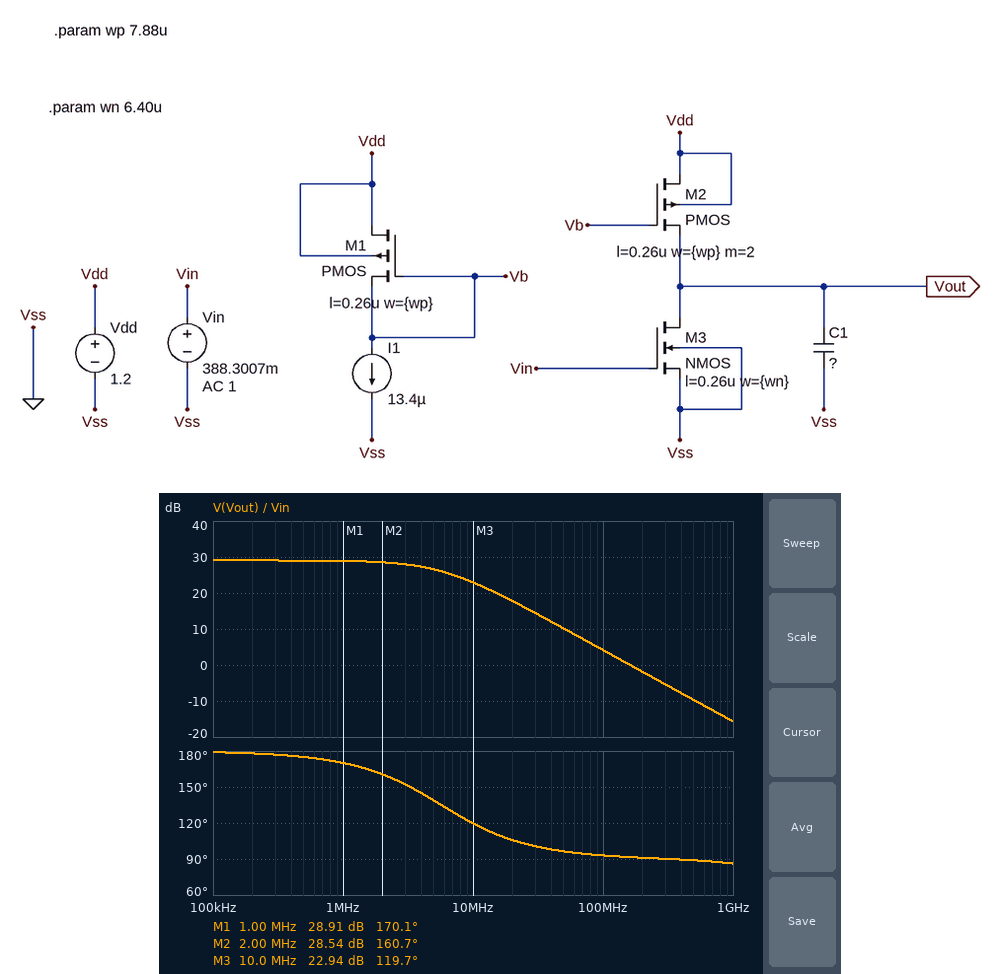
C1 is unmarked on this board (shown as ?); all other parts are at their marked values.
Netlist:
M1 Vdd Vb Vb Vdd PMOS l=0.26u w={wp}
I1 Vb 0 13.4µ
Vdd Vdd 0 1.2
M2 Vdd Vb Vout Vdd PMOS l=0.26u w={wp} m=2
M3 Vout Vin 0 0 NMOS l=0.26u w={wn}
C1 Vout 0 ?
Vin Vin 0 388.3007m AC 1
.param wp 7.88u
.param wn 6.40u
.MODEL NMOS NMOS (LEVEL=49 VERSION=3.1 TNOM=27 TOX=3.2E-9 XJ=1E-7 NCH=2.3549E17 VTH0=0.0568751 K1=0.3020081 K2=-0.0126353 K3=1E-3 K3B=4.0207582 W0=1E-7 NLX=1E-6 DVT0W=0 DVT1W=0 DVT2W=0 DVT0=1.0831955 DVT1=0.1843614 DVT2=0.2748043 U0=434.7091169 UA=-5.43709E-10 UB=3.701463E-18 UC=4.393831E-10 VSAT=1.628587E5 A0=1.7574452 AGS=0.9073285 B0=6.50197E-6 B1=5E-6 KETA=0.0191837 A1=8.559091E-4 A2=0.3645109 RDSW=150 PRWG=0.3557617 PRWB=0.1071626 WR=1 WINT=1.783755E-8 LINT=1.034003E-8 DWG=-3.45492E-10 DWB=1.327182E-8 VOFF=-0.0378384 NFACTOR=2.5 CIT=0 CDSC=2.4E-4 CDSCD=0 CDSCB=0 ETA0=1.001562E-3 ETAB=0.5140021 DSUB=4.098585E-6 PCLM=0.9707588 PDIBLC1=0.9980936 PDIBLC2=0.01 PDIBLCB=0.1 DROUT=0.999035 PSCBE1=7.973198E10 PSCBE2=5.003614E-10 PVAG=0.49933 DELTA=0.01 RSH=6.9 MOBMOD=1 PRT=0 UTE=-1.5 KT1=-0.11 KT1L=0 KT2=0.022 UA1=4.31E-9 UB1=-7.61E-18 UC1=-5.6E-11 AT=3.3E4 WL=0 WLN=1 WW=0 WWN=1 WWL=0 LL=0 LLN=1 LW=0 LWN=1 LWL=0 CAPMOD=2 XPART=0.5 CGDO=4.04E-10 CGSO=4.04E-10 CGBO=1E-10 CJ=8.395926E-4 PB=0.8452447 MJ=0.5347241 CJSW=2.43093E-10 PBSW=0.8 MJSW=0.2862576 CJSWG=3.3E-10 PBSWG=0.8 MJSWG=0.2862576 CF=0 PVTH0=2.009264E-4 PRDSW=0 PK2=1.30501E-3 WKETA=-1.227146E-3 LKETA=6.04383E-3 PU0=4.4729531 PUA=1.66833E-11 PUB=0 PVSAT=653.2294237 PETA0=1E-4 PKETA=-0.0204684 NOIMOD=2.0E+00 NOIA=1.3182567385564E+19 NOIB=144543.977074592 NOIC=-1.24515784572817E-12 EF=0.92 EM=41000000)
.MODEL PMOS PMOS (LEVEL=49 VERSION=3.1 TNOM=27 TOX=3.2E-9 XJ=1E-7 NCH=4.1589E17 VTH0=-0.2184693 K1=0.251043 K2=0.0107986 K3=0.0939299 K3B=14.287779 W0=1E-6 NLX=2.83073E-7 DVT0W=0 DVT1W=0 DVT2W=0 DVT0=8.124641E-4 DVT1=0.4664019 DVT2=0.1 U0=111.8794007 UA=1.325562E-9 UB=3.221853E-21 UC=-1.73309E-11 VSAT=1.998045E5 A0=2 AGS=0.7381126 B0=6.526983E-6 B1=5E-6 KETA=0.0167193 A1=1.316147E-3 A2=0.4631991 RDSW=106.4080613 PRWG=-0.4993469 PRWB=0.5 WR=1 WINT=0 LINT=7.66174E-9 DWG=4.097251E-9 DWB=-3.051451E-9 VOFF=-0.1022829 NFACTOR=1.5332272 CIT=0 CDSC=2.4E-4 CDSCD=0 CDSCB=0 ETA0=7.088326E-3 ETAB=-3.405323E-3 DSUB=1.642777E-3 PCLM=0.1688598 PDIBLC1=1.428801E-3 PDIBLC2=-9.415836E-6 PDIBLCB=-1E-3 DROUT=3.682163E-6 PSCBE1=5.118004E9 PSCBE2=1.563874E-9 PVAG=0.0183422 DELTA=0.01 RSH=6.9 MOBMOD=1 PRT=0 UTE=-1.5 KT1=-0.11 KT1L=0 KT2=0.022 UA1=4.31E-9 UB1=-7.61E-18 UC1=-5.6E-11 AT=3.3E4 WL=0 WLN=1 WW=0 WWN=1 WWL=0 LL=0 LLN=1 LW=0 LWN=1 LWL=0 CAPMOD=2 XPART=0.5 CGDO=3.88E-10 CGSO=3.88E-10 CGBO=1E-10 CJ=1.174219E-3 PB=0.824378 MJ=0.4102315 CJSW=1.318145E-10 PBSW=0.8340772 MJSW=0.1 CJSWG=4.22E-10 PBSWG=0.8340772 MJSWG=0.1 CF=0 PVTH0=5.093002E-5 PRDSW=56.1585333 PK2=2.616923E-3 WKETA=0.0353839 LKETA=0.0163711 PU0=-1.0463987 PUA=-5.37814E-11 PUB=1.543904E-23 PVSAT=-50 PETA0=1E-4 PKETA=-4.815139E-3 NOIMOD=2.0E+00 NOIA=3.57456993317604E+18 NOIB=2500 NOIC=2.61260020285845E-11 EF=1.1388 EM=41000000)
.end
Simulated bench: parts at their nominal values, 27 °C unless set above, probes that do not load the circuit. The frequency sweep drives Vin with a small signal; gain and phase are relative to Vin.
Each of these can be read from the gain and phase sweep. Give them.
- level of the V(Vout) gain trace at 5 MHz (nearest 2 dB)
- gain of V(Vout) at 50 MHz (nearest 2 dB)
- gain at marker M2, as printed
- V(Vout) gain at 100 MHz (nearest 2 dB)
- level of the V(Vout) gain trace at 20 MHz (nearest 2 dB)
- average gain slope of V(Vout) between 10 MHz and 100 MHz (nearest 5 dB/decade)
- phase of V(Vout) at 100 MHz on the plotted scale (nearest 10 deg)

26 dB
10 dB
28.54 dB
4 dB
18 dB
-20 dB/decade
90 deg
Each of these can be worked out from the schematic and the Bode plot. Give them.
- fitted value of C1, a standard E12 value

560 fF
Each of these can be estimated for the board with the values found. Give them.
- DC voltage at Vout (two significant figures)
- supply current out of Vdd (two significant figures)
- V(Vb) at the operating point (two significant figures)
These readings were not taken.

610 mV
42 µA
800 mV
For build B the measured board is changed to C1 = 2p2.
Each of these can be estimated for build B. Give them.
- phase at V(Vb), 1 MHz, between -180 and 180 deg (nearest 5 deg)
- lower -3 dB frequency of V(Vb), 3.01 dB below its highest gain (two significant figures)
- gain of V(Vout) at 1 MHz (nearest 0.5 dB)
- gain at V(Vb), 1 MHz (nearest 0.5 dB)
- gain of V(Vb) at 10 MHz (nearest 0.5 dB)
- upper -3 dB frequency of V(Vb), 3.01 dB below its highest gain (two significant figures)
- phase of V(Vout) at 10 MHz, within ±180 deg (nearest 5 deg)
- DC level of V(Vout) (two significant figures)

-125 deg
1.5 MHz
27.5 dB
-49.0 dB
-44.0 dB
620 MHz
100 deg
610 mV
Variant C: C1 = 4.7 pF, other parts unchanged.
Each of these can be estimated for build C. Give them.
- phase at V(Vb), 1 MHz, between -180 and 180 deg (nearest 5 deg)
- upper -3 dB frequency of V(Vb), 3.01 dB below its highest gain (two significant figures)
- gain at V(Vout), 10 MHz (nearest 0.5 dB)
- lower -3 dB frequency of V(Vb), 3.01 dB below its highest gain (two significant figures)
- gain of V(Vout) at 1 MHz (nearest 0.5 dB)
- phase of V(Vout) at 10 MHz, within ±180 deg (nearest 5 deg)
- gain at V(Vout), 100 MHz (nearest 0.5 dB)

-145 deg
620 MHz
6.0 dB
710 kHz
24.5 dB
95 deg
-14.0 dB
